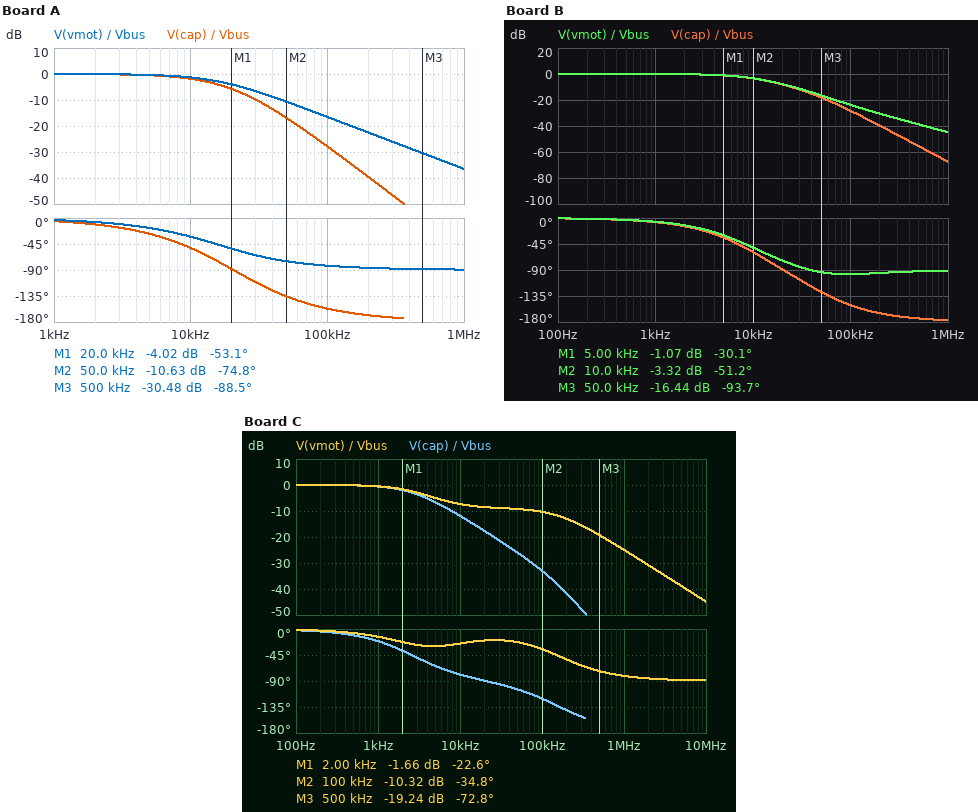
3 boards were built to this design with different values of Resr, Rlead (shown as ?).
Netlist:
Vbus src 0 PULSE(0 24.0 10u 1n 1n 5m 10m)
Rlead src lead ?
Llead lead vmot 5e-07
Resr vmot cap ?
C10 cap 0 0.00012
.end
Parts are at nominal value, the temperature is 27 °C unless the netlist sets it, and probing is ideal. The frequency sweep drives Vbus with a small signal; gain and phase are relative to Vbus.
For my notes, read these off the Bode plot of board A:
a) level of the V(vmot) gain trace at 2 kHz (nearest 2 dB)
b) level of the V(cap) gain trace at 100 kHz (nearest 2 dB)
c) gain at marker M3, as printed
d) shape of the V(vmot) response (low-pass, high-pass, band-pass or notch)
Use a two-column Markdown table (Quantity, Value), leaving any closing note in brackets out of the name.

| Quantity | Value |
|---|---|
| level of the V(vmot) gain trace at 2 kHz | 0 dB |
| level of the V(cap) gain trace at 100 kHz | -28 dB |
| gain at marker M3, as printed | -30.48 dB |
| shape of the V(vmot) response | low-pass |
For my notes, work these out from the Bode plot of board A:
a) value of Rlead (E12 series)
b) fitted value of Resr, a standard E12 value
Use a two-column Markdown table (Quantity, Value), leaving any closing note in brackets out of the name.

| Quantity | Value |
|---|---|
| value of Rlead | 0.082 Ω |
| fitted value of Resr, a standard E12 value | 0.047 Ω |
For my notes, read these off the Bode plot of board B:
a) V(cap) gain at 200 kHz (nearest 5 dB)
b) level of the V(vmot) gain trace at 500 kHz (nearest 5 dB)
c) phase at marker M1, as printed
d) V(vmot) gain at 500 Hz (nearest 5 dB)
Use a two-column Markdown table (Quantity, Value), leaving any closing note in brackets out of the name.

| Quantity | Value |
|---|---|
| V(cap) gain at 200 kHz | -40 dB |
| level of the V(vmot) gain trace at 500 kHz | -40 dB |
| phase at marker M1, as printed | -30.1 deg |
| V(vmot) gain at 500 Hz | 0 dB |
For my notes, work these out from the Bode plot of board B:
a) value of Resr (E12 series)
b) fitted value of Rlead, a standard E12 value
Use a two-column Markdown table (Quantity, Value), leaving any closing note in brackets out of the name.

| Quantity | Value |
|---|---|
| value of Resr | 0.018 Ω |
| fitted value of Rlead, a standard E12 value | 0.15 Ω |
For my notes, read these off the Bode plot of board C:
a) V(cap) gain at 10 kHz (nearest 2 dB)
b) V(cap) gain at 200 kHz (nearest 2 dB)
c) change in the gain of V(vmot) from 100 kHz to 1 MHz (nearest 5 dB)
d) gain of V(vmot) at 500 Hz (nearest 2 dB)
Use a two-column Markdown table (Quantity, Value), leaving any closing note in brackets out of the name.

| Quantity | Value |
|---|---|
| V(cap) gain at 10 kHz | -12 dB |
| V(cap) gain at 200 kHz | -42 dB |
| change in the gain of V(vmot) from 100 kHz to 1 MHz | -15 dB |
| gain of V(vmot) at 500 Hz | 0 dB |
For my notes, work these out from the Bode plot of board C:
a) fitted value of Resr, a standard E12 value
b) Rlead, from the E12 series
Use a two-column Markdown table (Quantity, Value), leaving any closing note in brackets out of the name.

| Quantity | Value |
|---|---|
| fitted value of Resr, a standard E12 value | 0.18 Ω |
| Rlead, from the E12 series | 0.33 Ω |
